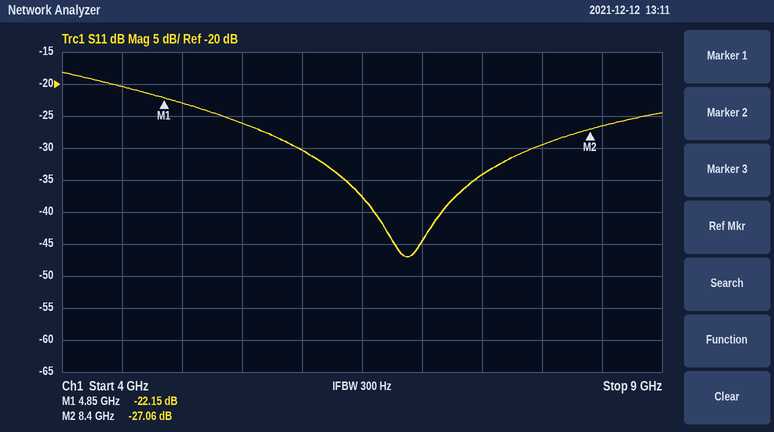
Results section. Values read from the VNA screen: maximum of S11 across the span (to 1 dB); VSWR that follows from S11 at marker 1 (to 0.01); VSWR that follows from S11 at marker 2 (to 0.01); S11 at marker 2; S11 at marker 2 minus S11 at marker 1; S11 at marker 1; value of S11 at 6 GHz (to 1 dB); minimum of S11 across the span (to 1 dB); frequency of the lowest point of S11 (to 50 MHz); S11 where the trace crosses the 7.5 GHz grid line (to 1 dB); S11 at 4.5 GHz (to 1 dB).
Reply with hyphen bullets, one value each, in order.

- -18 dB
- 1.17
- 1.09
- -27.06 dB
- -4.91 dB
- -22.15 dB
- -30 dB
- -47 dB
- 6.85 GHz
- -34 dB
- -20 dB
